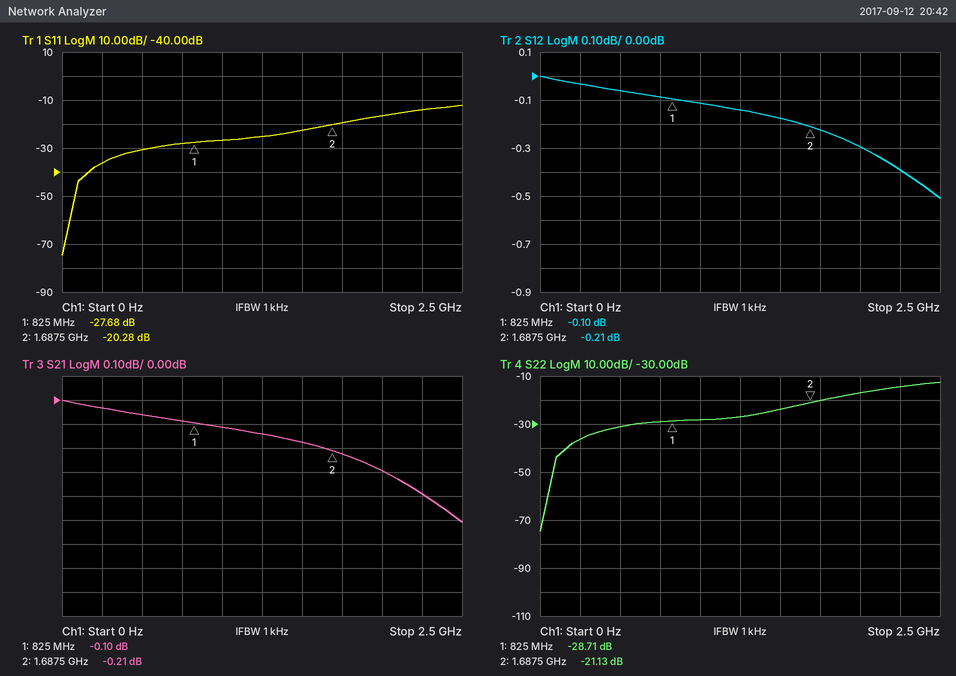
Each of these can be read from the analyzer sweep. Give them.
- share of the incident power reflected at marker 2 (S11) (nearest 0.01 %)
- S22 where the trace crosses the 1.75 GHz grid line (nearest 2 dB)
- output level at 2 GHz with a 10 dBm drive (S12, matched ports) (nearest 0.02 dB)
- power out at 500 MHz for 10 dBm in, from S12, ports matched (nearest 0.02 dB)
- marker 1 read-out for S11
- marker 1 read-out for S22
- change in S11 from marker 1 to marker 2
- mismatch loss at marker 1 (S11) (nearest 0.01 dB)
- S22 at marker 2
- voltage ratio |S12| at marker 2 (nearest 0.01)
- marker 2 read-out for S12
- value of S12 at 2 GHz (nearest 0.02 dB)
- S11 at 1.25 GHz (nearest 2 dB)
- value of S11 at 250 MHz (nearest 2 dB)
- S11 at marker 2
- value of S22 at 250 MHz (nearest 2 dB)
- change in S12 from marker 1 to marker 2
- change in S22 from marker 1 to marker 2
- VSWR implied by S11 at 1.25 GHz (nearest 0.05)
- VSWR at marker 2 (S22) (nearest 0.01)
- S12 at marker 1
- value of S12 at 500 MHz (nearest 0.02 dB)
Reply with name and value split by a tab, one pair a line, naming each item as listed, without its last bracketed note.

share of the incident power reflected at marker 2 (S11)	0.94 %
S22 where the trace crosses the 1.75 GHz grid line	-20 dB
output level at 2 GHz with a 10 dBm drive (S12, matched ports)	9.70 dBm
power out at 500 MHz for 10 dBm in, from S12, ports matched	9.94 dBm
marker 1 read-out for S11	-27.68 dB
marker 1 read-out for S22	-28.71 dB
change in S11 from marker 1 to marker 2	7.40 dB
mismatch loss at marker 1 (S11)	0.01 dB
S22 at marker 2	-21.13 dB
voltage ratio |S12| at marker 2	0.98
marker 2 read-out for S12	-0.21 dB
value of S12 at 2 GHz	-0.30 dB
S11 at 1.25 GHz	-26 dB
value of S11 at 250 MHz	-36 dB
S11 at marker 2	-20.28 dB
value of S22 at 250 MHz	-36 dB
change in S12 from marker 1 to marker 2	-0.11 dB
change in S22 from marker 1 to marker 2	7.58 dB
VSWR implied by S11 at 1.25 GHz	1.10
VSWR at marker 2 (S22)	1.19
S12 at marker 1	-0.10 dB
value of S12 at 500 MHz	-0.06 dB
